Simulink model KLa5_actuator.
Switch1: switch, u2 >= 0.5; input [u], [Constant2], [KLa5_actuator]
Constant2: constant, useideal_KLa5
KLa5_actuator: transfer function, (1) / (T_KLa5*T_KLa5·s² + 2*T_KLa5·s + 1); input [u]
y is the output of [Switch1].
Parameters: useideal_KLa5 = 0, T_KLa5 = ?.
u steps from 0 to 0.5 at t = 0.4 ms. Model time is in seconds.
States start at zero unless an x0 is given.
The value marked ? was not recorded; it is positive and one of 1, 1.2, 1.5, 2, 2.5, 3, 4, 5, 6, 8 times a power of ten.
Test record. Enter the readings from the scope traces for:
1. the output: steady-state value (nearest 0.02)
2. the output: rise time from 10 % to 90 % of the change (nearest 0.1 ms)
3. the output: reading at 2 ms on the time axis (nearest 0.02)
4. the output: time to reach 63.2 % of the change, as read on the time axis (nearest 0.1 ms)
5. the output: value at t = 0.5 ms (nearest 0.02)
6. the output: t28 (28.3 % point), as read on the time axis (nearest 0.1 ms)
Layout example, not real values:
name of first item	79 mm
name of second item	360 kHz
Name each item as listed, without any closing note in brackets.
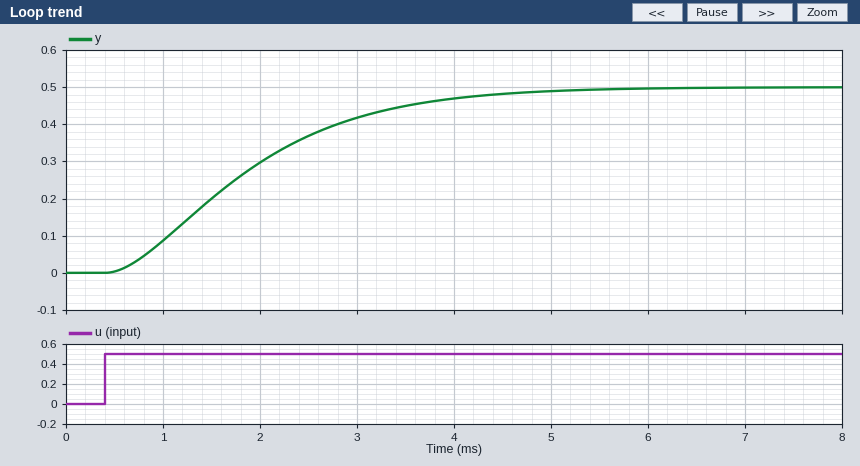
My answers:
the output: steady-state value	0.50
the output: rise time from 10 % to 90 % of the change	2.7 ms
the output: reading at 2 ms on the time axis	0.30
the output: time to reach 63.2 % of the change, as read on the time axis	2.1 ms
the output: value at t = 0.5 ms	0.00
the output: t28 (28.3 % point), as read on the time axis	1.2 ms
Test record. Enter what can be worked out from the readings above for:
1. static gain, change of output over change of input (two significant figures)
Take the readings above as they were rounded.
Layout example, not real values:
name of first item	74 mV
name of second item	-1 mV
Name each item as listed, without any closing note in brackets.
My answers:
static gain, change of output over change of input	1.0
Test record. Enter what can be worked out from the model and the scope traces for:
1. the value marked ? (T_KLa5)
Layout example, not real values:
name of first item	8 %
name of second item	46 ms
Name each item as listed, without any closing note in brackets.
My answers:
the value marked ?	0.0008
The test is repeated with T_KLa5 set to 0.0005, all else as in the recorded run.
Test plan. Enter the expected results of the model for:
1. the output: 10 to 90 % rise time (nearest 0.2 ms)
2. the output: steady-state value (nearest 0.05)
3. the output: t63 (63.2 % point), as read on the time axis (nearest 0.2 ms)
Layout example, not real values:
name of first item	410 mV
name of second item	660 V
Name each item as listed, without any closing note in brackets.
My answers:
the output: 10 to 90 % rise time	1.6 ms
the output: steady-state value	0.50
the output: t63 (63.2 % point), as read on the time axis	1.4 ms
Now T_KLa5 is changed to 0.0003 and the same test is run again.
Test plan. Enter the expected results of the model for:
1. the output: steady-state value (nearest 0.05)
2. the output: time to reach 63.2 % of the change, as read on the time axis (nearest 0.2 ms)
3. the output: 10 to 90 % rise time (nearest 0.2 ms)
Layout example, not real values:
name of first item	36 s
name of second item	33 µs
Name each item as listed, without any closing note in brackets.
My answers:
the output: steady-state value	0.50
the output: time to reach 63.2 % of the change, as read on the time axis	1.0 ms
the output: 10 to 90 % rise time	1.0 ms
